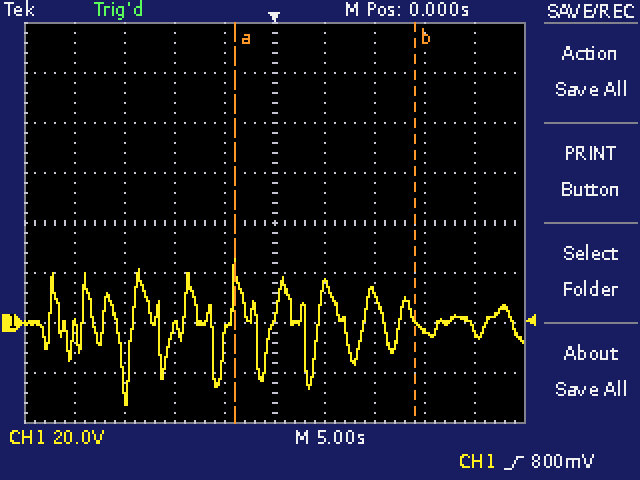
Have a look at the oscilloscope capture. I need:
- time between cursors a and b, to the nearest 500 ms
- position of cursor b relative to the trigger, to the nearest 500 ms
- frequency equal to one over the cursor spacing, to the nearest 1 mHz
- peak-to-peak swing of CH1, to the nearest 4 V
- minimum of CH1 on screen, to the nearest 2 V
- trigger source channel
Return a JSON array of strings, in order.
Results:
["18.0 s", "+14.0 s", "56 mHz", "60 V", "-32 V", "CH1"]
